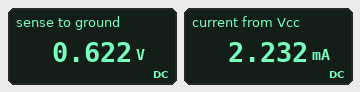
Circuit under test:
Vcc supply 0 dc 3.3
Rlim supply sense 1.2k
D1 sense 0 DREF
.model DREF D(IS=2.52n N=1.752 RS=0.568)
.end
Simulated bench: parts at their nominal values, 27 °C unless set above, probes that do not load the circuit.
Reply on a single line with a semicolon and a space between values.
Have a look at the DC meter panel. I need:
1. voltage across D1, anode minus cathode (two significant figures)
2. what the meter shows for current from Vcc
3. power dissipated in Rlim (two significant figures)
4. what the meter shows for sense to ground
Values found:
620 mV; 2.232 mA; 6.0 mW; 0.622 V
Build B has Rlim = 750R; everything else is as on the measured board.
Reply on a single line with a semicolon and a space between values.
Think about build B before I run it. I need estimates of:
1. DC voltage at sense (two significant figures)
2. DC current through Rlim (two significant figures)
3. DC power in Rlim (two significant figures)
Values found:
640 mV; 3.5 mA; 9.4 mW
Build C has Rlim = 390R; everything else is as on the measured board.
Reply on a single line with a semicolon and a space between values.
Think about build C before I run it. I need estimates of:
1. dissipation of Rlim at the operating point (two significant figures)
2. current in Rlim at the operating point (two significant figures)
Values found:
18 mW; 6.7 mA
